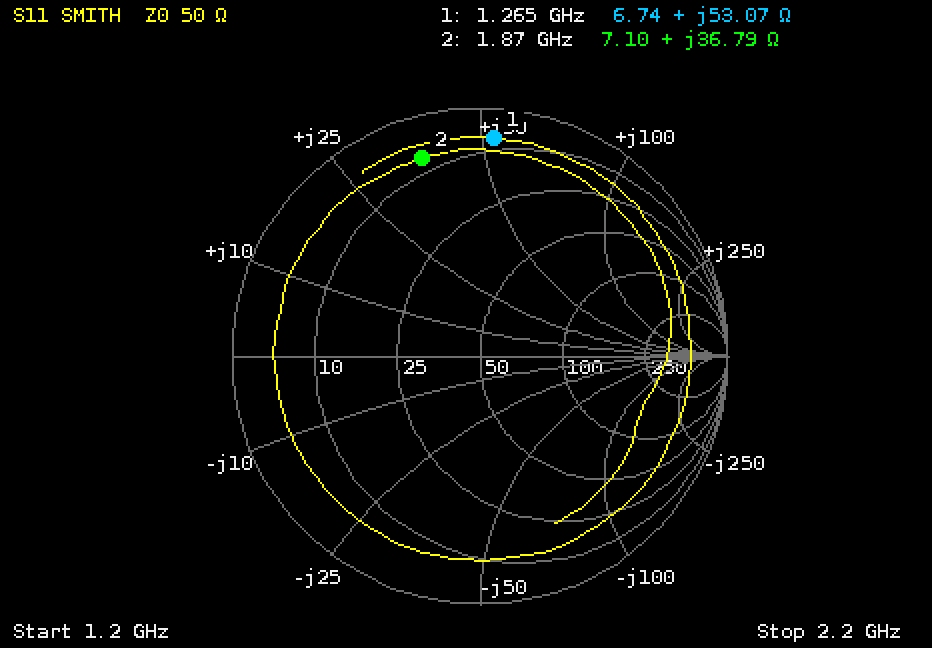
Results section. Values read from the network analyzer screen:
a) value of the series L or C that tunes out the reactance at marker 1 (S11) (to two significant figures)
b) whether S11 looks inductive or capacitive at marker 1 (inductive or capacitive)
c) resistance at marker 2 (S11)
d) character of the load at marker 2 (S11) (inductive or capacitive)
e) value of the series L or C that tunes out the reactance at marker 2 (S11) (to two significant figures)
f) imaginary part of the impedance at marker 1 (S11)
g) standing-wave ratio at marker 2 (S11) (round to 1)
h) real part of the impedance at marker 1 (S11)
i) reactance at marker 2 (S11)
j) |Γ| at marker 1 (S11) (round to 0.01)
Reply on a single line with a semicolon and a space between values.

2.4 pF; inductive; 7.10 Ω; inductive; 2.3 pF; +53.07 Ω; 11; 6.74 Ω; +36.79 Ω; 0.88
